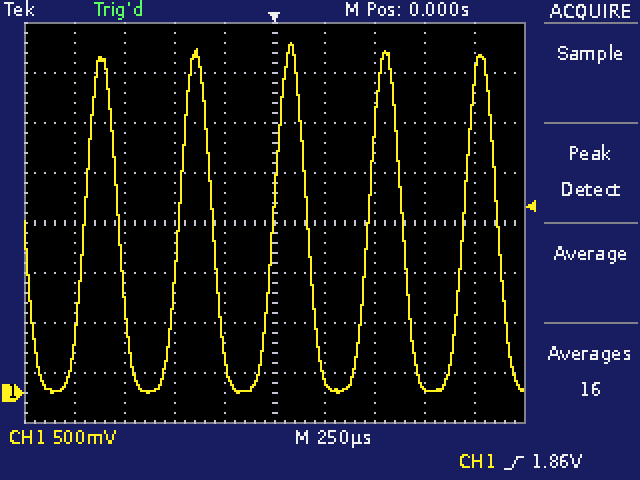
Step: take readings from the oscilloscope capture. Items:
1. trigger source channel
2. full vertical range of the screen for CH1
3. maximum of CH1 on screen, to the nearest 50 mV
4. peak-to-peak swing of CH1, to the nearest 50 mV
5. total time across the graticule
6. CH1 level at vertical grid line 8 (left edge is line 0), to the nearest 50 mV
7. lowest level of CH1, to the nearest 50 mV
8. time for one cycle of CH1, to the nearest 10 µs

CH1
4 V
3.50 V
3.50 V
2.5 ms
50 mV
0 mV
470 µs
